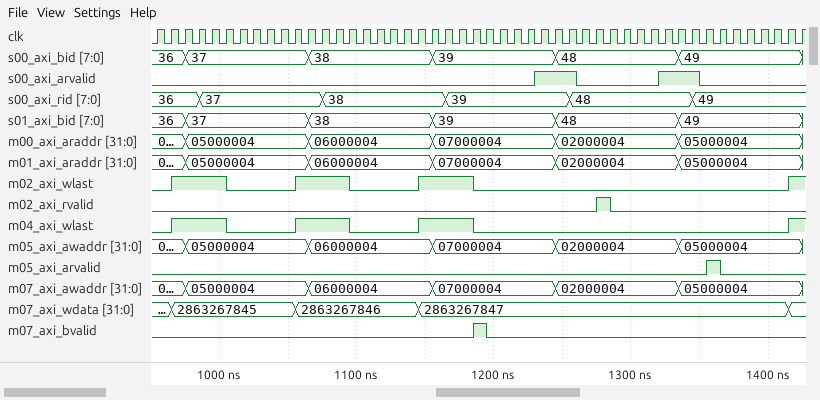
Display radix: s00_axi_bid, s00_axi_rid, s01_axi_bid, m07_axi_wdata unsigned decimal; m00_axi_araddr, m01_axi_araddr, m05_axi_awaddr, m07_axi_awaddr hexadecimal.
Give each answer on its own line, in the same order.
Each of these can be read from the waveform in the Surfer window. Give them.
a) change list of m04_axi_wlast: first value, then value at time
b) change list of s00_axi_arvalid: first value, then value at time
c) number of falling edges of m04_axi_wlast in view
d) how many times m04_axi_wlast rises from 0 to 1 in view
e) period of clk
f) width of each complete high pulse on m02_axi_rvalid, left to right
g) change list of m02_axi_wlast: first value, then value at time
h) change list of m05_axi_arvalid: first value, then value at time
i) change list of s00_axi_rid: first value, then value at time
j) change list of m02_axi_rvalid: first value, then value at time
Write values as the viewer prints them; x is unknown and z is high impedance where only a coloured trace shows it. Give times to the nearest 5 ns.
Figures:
0, 1 at 965 ns, 0 at 1005 ns, 1 at 1055 ns, 0 at 1095 ns, 1 at 1145 ns, 0 at 1185 ns, 1 at 1415 ns
0, 1 at 1230 ns, 0 at 1260 ns, 1 at 1320 ns, 0 at 1350 ns
3
4
10 ns
10 ns
0, 1 at 965 ns, 0 at 1005 ns, 1 at 1055 ns, 0 at 1095 ns, 1 at 1145 ns, 0 at 1185 ns, 1 at 1415 ns
0, 1 at 1355 ns, 0 at 1365 ns
36, 37 at 985 ns, 38 at 1075 ns, 39 at 1165 ns, 48 at 1255 ns, 49 at 1345 ns
0, 1 at 1275 ns, 0 at 1285 ns
